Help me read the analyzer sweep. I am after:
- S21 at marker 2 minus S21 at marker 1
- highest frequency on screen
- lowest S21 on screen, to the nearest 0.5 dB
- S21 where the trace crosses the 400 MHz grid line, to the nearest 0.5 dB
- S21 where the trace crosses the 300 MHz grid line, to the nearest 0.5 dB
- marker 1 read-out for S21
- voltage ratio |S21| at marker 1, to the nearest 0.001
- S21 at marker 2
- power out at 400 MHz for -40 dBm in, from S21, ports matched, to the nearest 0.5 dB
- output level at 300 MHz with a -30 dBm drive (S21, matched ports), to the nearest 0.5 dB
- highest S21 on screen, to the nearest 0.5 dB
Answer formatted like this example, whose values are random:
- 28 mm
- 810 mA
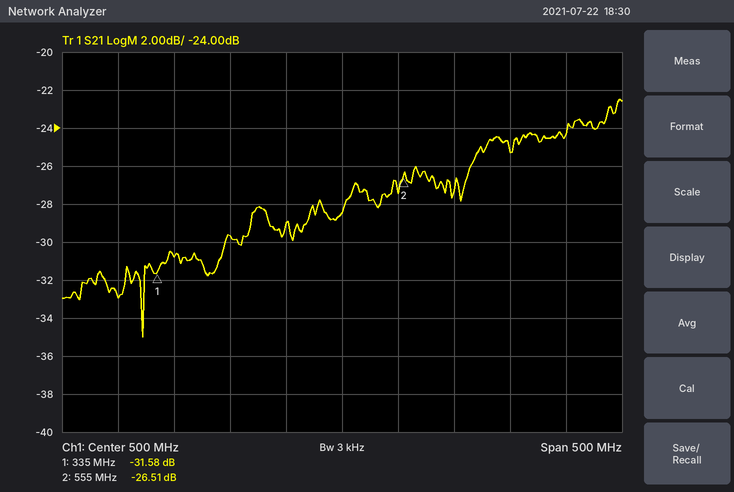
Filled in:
- 5.07 dB
- 750 MHz
- -35.0 dB
- -29.5 dB
- -33.0 dB
- -31.58 dB
- 0.026
- -26.51 dB
- -69.5 dBm
- -63.0 dBm
- -22.5 dB
